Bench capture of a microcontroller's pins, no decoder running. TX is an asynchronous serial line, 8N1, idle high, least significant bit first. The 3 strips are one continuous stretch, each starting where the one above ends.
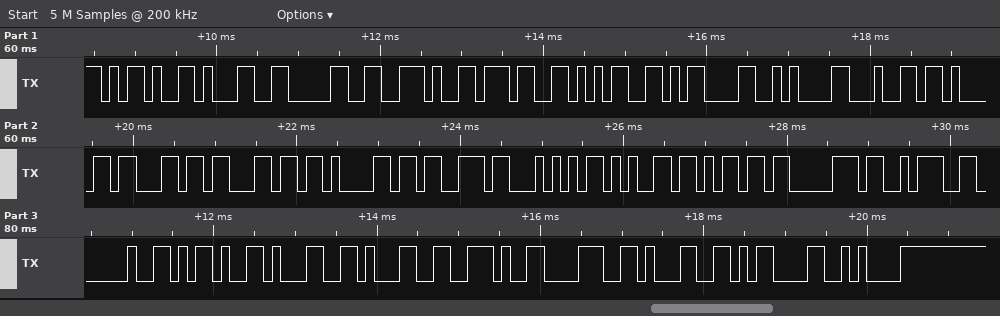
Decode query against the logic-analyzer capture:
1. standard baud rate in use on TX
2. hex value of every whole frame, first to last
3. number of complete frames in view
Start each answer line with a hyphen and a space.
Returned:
- 9600 baud
- 0x2D 0x31 0x30 0x2E 0x37 0x35 0x0D 0x0A 0x64 0x61 0x6C 0x6C 0x61 0x73 0x54 0x65 0x6D 0x70 0x3A 0x20 0x2D 0x31 0x31 0x2E 0x38 0x31 0x0D 0x0A
- 28
